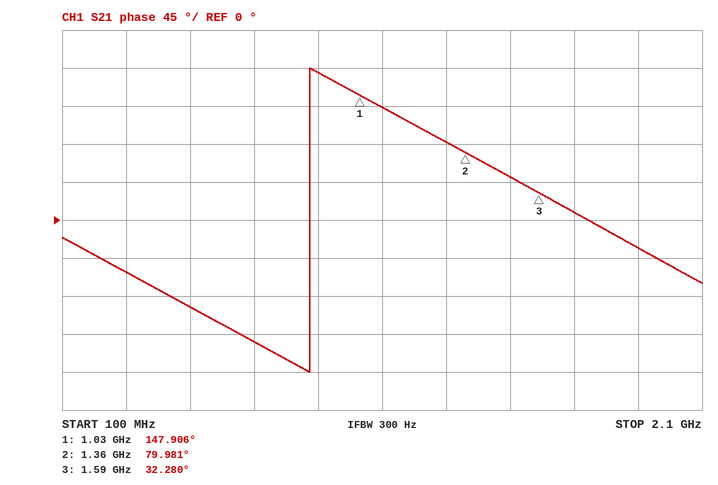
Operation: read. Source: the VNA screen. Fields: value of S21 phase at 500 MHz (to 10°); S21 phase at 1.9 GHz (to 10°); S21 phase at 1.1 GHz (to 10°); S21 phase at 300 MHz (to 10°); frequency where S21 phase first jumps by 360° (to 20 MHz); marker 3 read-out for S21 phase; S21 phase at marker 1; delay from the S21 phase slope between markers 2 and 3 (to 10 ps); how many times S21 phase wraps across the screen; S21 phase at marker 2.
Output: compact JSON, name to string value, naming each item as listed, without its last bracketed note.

{"value of S21 phase at 500 MHz": "-100°", "S21 phase at 1.9 GHz": "-30°", "S21 phase at 1.1 GHz": "130°", "S21 phase at 300 MHz": "-60°", "frequency where S21 phase first jumps by 360°": "880 MHz", "marker 3 read-out for S21 phase": "32.280°", "S21 phase at marker 1": "147.906°", "delay from the S21 phase slope between markers 2 and 3": "580 ps", "how many times S21 phase wraps across the screen": "1", "S21 phase at marker 2": "79.981°"}
